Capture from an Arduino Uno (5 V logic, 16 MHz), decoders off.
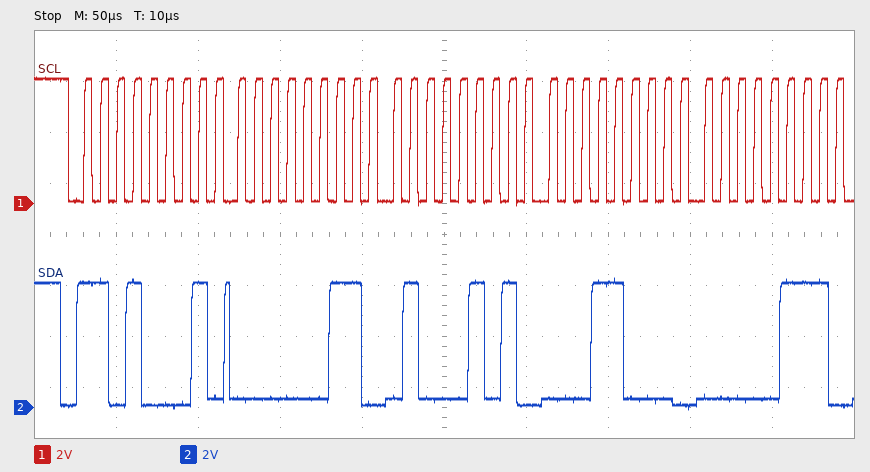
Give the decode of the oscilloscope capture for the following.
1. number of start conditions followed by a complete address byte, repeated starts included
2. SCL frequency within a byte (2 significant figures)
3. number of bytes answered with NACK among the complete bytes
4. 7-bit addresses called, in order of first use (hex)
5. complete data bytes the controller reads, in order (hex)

1
100 kHz
0
0x68
03 45 18 07
